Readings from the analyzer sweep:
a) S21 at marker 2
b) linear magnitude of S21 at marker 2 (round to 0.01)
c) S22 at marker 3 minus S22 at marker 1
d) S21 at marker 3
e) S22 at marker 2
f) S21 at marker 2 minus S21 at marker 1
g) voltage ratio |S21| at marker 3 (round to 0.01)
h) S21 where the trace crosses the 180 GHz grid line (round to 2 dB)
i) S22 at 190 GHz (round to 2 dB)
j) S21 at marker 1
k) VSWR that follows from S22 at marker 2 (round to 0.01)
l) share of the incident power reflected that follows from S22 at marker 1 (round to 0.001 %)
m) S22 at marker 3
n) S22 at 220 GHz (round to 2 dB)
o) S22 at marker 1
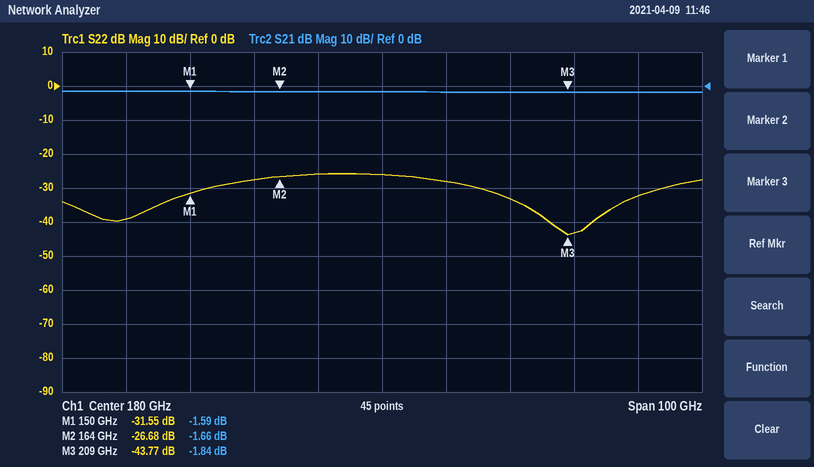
-1.66 dB
0.83
-12.22 dB
-1.84 dB
-26.68 dB
-0.07 dB
0.81
-2 dB
-28 dB
-1.59 dB
1.10
0.070 %
-43.77 dB
-32 dB
-31.55 dB
